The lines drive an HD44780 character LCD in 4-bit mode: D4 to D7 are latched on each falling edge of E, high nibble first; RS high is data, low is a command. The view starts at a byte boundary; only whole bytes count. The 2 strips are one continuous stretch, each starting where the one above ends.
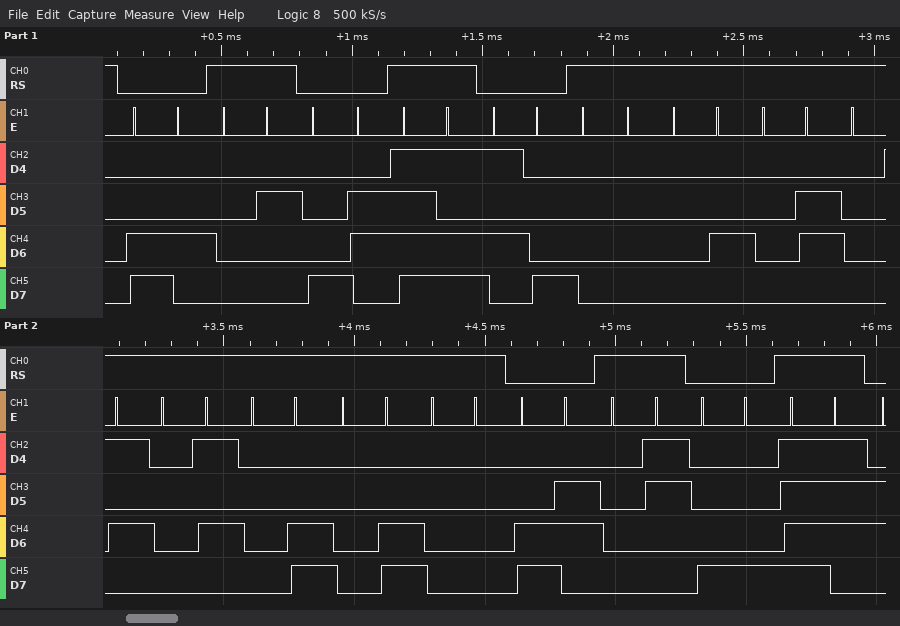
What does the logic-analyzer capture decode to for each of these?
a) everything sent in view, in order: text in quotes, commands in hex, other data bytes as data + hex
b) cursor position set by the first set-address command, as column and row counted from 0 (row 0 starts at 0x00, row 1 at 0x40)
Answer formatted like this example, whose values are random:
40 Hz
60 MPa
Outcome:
0xC4 data 02 0x86 data FD 0x58 data 00 04 06 05 05 0C 0C 00 0xC6 data 03 0x88 data F7
column 4, row 1
